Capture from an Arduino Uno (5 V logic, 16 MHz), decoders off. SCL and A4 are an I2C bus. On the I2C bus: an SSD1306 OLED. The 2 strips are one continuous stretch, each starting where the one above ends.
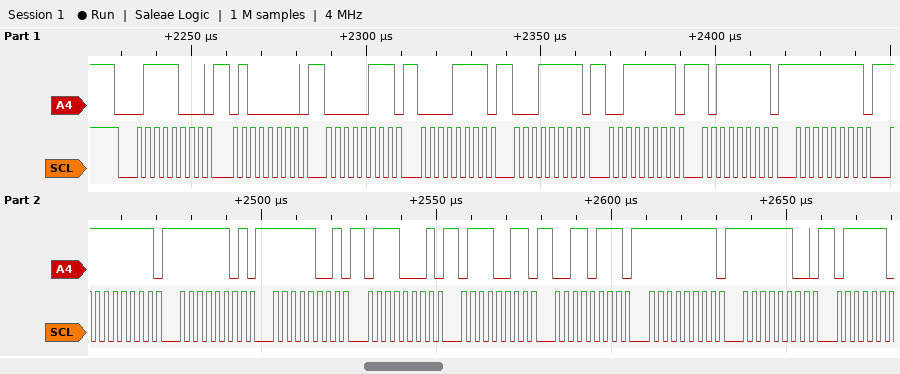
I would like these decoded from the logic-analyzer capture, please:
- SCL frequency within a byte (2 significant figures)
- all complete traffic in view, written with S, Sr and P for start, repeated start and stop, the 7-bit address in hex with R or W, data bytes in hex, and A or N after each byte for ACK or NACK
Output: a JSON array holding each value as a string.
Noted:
["400 kHz", "S 3CW A 40 A 07 A 0F A 1F A 3F A BF A FF A FF A FD A F9 A 71 A 73 A 37 A FF A FC A"]
